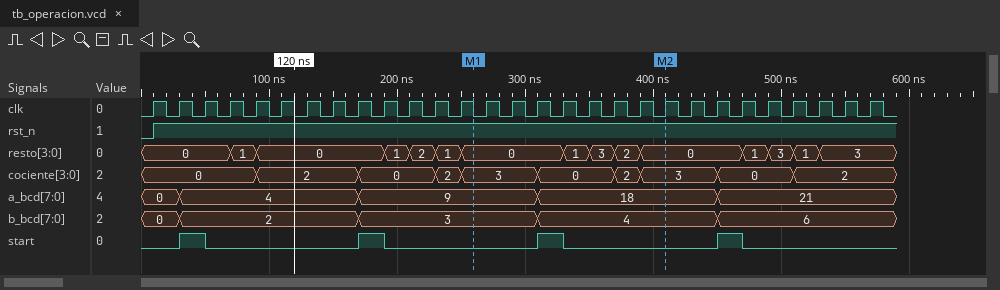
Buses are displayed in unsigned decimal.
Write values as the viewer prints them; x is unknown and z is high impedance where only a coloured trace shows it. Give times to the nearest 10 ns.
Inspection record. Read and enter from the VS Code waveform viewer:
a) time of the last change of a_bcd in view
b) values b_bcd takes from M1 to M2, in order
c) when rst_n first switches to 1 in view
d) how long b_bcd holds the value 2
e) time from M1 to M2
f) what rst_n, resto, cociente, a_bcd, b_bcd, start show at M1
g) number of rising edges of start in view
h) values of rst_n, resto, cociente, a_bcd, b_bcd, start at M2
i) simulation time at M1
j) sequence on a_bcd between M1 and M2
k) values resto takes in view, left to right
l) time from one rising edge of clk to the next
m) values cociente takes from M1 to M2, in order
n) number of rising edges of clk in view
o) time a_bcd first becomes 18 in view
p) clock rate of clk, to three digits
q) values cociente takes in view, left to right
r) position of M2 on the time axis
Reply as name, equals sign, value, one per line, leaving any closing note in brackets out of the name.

time of the last change of a_bcd in view = 450 ns
values b_bcd takes from M1 to M2, in order = 3, 4
when rst_n first switches to 1 in view = 10 ns
how long b_bcd holds the value 2 = 140 ns
time from M1 to M2 = 150 ns
what rst_n, resto, cociente, a_bcd, b_bcd, start show at M1 = rst_n=1, resto=0, cociente=3, a_bcd=9, b_bcd=3, start=0
number of rising edges of start in view = 4
values of rst_n, resto, cociente, a_bcd, b_bcd, start at M2 = rst_n=1, resto=0, cociente=3, a_bcd=18, b_bcd=4, start=0
simulation time at M1 = 260 ns
sequence on a_bcd between M1 and M2 = 9, 18
values resto takes in view, left to right = 0, 1, 0, 1, 2, 1, 0, 1, 3, 2, 0, 1, 3, 1, 3
time from one rising edge of clk to the next = 20 ns
values cociente takes from M1 to M2, in order = 3, 0, 2, 3
number of rising edges of clk in view = 29
time a_bcd first becomes 18 in view = 310 ns
clock rate of clk, to three digits = 50.0 MHz
values cociente takes in view, left to right = 0, 2, 0, 2, 3, 0, 2, 3, 0, 2
position of M2 on the time axis = 410 ns
